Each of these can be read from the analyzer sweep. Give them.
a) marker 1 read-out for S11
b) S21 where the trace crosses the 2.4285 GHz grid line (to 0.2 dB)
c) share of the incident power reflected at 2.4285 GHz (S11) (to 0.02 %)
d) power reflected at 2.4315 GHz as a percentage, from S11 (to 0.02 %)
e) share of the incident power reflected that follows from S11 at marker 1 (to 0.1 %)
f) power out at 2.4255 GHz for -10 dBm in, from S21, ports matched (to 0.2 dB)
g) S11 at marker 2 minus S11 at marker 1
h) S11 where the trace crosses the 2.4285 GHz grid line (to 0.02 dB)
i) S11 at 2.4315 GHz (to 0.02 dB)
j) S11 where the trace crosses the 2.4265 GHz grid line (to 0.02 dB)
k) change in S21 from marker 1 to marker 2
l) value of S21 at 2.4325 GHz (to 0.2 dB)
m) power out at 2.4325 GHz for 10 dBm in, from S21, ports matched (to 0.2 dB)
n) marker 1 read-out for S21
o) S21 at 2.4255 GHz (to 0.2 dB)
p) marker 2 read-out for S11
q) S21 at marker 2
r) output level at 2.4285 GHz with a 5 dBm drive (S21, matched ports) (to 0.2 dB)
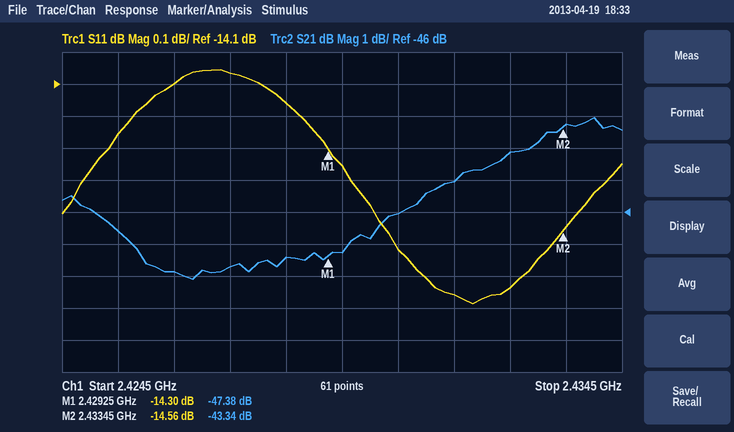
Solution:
-14.30 dB
-47.4 dB
3.84 %
3.34 %
3.7 %
-56.6 dBm
-0.26 dB
-14.16 dB
-14.76 dB
-14.10 dB
4.04 dB
-44.2 dB
-34.2 dBm
-47.38 dB
-46.6 dB
-14.56 dB
-43.34 dB
-42.4 dBm
